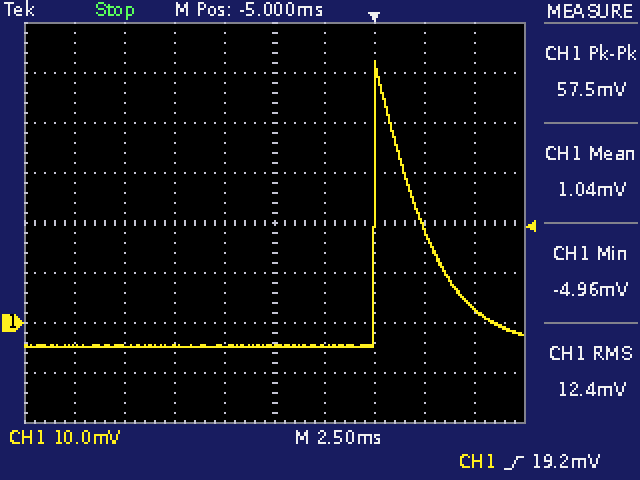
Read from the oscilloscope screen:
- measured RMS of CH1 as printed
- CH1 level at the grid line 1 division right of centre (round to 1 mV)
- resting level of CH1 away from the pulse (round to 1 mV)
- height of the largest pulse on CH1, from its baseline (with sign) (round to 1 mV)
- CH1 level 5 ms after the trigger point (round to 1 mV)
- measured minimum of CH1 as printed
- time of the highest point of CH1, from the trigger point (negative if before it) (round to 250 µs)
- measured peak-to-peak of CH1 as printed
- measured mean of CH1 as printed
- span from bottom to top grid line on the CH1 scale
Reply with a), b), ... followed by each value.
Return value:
a) 12.4 mV
b) -5 mV
c) -5 mV
d) +57 mV
e) 3 mV
f) -4.96 mV
g) 0.00 ms
h) 57.5 mV
i) 1.04 mV
j) 80 mV
